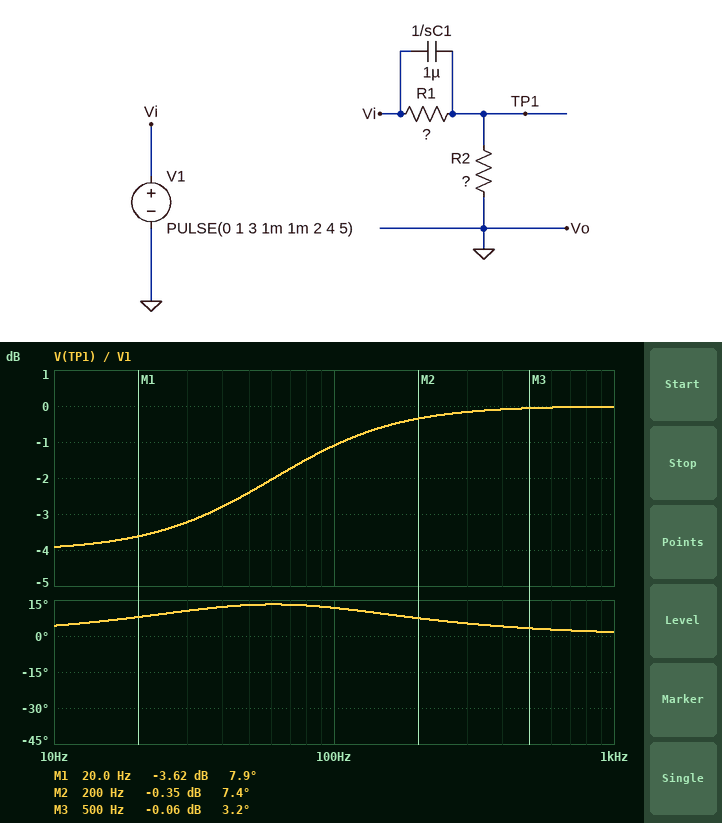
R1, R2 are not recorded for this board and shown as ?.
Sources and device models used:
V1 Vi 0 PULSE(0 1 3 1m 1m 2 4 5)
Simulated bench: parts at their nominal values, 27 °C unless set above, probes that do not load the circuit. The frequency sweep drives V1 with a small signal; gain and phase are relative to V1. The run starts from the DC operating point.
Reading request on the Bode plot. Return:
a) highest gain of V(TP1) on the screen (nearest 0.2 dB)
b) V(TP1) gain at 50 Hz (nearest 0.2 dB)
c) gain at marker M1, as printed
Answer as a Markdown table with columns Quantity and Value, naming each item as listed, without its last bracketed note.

| Quantity | Value |
|---|---|
| highest gain of V(TP1) on the screen | 0 dB |
| V(TP1) gain at 50 Hz | -2.4 dB |
| gain at marker M1, as printed | -3.62 dB |
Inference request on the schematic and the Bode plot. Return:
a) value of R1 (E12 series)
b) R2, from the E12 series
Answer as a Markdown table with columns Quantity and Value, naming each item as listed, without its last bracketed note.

| Quantity | Value |
|---|---|
| value of R1 | 3.3 kΩ |
| R2, from the E12 series | 5.6 kΩ |
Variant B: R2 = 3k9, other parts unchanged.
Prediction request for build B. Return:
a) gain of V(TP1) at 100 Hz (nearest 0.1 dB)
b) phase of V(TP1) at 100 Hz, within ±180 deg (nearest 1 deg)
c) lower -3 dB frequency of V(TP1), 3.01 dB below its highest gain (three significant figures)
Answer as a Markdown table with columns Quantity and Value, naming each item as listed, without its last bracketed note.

| Quantity | Value |
|---|---|
| gain of V(TP1) at 100 Hz | -1.6 dB |
| phase of V(TP1) at 100 Hz, within ±180 deg | 16 deg |
| lower -3 dB frequency of V(TP1), 3.01 dB below its highest gain | 57.2 Hz |
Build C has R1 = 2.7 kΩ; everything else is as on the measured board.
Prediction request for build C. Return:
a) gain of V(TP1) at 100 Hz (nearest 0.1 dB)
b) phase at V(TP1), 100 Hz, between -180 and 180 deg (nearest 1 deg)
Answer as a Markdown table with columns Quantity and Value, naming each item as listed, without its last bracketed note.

| Quantity | Value |
|---|---|
| gain of V(TP1) at 100 Hz | -1.2 dB |
| phase at V(TP1), 100 Hz, between -180 and 180 deg | 11 deg |
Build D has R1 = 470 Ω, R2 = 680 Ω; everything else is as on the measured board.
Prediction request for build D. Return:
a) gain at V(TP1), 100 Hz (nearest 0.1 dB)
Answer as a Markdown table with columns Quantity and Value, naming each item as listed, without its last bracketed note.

| Quantity | Value |
|---|---|
| gain at V(TP1), 100 Hz | -4.3 dB |
